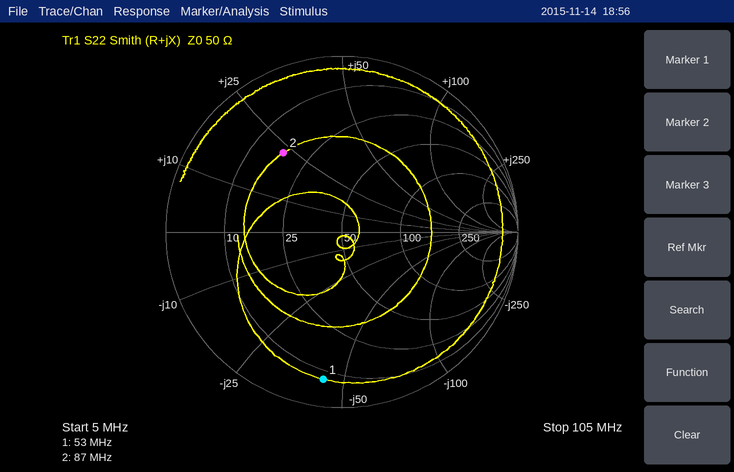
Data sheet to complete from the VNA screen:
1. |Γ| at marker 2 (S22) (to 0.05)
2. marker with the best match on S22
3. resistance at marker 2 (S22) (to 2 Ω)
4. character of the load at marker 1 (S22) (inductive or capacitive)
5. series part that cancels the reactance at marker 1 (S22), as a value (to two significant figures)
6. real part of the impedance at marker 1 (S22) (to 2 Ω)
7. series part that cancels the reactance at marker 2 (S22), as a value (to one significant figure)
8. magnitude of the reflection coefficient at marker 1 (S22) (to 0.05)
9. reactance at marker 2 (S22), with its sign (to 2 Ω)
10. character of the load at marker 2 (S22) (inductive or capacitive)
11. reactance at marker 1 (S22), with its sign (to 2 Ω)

0.55
marker 2
18 Ω
capacitive
130 nH
8 Ω
80 pF
0.85
+22 Ω
inductive
-44 Ω
